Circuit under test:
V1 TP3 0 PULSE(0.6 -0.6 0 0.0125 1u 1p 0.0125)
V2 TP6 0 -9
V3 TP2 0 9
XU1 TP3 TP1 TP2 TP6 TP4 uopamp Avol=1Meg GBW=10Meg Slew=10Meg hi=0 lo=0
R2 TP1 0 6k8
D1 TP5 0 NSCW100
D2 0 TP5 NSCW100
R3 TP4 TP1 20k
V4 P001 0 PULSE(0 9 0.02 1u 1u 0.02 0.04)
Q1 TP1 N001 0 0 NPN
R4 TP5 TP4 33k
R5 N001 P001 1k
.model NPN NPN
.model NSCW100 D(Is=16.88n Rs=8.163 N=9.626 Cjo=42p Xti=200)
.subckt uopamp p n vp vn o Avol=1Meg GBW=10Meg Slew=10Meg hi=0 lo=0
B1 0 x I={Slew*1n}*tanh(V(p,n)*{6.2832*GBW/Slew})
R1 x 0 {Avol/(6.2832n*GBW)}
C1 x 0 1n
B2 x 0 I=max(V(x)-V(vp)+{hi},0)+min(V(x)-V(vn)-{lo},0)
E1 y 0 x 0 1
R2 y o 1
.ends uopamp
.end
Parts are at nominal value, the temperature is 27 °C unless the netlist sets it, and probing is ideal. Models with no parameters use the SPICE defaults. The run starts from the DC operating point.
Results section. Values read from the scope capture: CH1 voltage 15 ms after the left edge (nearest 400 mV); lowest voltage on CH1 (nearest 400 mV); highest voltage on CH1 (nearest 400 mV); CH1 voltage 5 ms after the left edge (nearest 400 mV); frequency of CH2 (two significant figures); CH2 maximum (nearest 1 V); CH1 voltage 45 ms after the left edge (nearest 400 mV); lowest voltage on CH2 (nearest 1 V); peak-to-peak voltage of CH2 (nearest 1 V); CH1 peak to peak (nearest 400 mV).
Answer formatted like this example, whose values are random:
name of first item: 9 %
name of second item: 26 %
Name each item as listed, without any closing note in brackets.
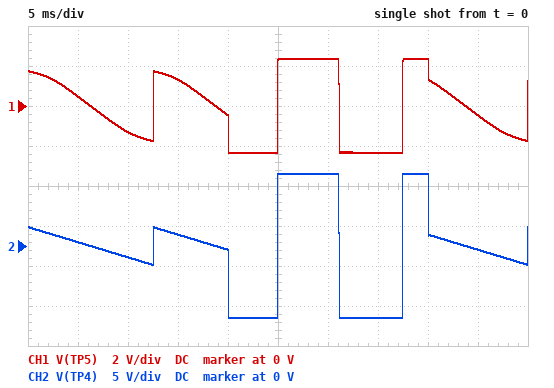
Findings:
CH1 voltage 15 ms after the left edge: 1.2 V
lowest voltage on CH1: -2.4 V
highest voltage on CH1: 2.4 V
CH1 voltage 5 ms after the left edge: 400 mV
frequency of CH2: 80 Hz
CH2 maximum: 9 V
CH1 voltage 45 ms after the left edge: -400 mV
lowest voltage on CH2: -9 V
peak-to-peak voltage of CH2: 18 V
CH1 peak to peak: 4.8 V
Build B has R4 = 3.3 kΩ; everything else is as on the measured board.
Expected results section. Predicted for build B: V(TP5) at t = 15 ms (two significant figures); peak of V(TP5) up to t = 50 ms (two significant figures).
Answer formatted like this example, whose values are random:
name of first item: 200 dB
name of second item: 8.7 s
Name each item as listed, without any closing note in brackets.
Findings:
V(TP5) at t = 15 ms: 1.4 V
peak of V(TP5) up to t = 50 ms: 2.9 V
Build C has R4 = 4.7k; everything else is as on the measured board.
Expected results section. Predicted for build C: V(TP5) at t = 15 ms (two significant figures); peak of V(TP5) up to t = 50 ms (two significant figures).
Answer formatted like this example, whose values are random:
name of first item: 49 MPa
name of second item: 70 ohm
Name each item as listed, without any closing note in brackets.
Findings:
V(TP5) at t = 15 ms: 1.4 V
peak of V(TP5) up to t = 50 ms: 2.8 V
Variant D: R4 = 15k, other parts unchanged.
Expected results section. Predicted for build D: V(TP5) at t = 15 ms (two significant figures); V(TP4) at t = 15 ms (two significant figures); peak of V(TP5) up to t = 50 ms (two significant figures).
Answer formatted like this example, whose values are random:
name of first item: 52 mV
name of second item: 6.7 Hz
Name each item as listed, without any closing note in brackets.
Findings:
V(TP5) at t = 15 ms: 1.4 V
V(TP4) at t = 15 ms: 1.4 V
peak of V(TP5) up to t = 50 ms: 2.5 V
